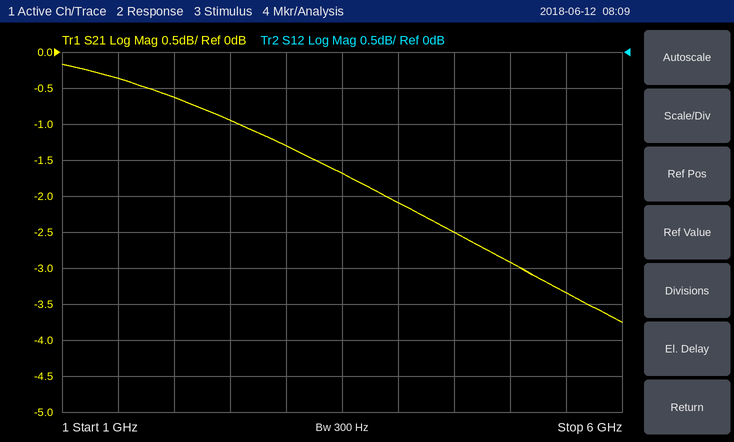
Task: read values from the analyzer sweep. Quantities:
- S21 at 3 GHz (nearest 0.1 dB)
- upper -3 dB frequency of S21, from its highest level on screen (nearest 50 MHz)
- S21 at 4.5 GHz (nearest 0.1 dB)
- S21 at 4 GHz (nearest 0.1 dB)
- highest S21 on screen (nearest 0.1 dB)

-1.3 dB
5.30 GHz
-2.5 dB
-2.1 dB
-0.2 dB
